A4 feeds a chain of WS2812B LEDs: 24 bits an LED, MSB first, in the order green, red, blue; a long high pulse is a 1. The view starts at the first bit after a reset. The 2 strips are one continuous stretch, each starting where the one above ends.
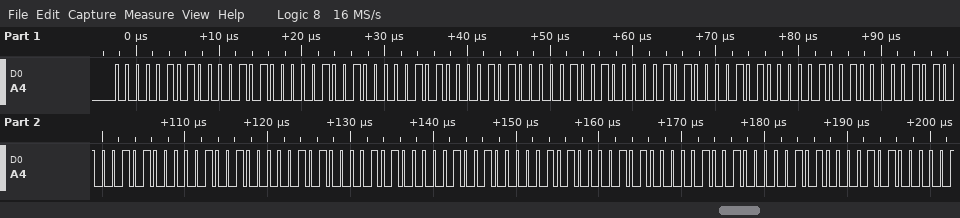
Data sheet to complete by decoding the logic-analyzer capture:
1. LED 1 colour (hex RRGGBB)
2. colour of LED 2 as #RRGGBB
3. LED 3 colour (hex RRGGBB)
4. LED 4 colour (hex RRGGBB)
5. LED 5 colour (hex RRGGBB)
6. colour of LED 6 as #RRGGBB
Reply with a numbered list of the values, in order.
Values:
1. #0A0509
2. #0A0509
3. #0A0509
4. #0A0509
5. #0A0509
6. #0A0509
